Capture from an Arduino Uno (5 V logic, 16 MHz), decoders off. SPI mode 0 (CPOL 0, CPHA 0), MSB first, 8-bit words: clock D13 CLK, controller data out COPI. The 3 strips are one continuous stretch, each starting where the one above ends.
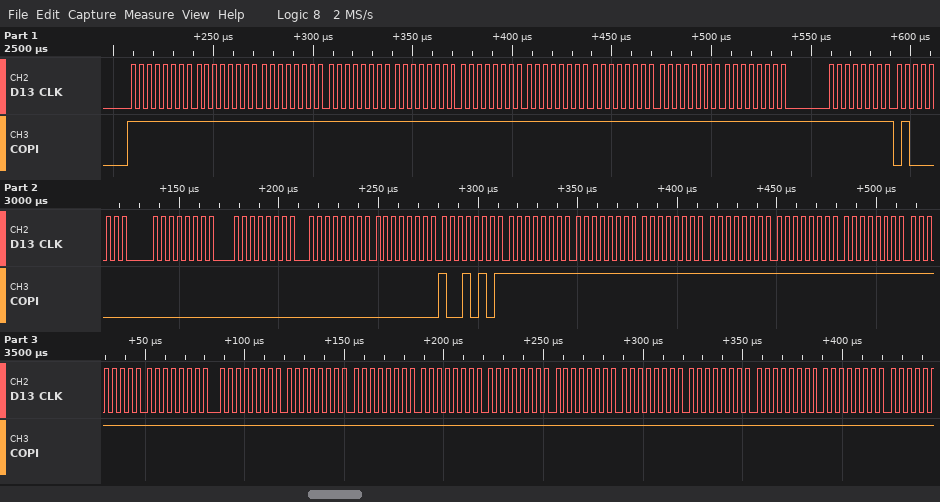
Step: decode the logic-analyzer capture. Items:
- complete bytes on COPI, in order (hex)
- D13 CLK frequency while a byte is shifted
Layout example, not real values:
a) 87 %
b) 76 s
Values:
a) 0xFF 0xFF 0xFF 0xFF 0xFF 0xFF 0xFF 0xFF 0xFF 0xFF 0xFF 0x40 0x00 0x00 0x00 0x00 0x95 0xFF 0xFF 0xFF 0xFF 0xFF 0xFF 0xFF 0xFF 0xFF 0xFF 0xFF 0xFF 0xFF 0xFF 0xFF 0xFF 0xFF 0xFF
b) 250 kHz
